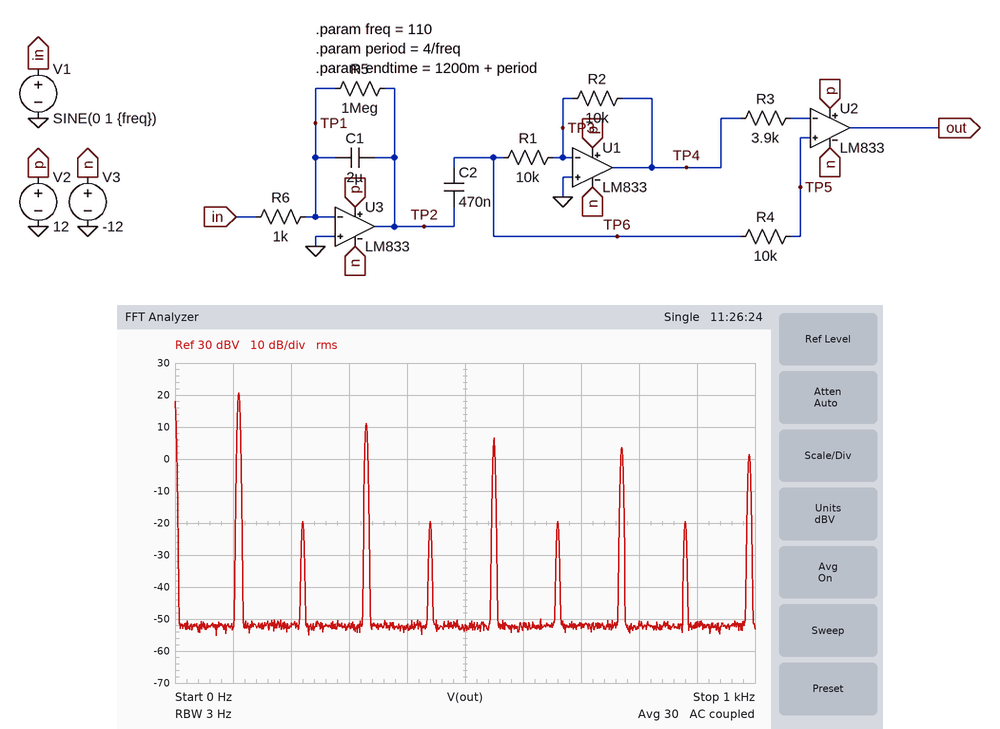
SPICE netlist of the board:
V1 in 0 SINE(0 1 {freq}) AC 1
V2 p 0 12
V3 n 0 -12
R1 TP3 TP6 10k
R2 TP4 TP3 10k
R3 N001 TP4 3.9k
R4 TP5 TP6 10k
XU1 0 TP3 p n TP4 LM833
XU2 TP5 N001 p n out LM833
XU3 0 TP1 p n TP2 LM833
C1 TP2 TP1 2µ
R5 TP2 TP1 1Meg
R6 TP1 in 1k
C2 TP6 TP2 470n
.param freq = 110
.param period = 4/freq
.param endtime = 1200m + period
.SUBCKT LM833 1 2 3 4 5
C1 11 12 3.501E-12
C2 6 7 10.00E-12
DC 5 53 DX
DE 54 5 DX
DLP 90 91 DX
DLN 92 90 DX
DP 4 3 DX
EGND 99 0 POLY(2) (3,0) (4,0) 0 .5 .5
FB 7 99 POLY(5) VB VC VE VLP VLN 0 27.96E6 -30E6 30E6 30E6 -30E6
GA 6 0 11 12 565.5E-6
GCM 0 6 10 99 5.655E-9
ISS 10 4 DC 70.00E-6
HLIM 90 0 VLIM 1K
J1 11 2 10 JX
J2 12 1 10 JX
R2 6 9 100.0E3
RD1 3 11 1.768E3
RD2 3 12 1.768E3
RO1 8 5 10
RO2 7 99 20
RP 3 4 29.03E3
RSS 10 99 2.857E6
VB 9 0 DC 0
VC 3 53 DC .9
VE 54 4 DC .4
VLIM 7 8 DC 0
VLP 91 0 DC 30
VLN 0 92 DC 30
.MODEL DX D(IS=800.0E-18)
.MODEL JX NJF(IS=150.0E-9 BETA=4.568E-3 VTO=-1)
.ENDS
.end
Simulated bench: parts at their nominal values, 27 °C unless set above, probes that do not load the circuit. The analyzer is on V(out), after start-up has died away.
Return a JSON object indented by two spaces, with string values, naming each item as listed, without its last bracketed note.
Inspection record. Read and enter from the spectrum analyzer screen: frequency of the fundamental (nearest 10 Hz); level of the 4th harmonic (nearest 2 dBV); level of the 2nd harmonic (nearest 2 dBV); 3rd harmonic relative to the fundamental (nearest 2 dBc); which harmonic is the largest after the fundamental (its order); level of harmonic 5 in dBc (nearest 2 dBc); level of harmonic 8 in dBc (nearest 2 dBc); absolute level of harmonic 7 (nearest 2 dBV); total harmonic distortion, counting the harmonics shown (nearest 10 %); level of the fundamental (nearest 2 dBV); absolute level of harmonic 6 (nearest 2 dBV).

{
  "frequency of the fundamental": "110 Hz",
  "level of the 4th harmonic": "-20 dBV",
  "level of the 2nd harmonic": "-20 dBV",
  "3rd harmonic relative to the fundamental": "-10 dBc",
  "which harmonic is the largest after the fundamental": "3",
  "level of harmonic 5 in dBc": "-14 dBc",
  "level of harmonic 8 in dBc": "-40 dBc",
  "absolute level of harmonic 7": "4 dBV",
  "total harmonic distortion, counting the harmonics shown": "40 %",
  "level of the fundamental": "20 dBV",
  "absolute level of harmonic 6": "-20 dBV"
}
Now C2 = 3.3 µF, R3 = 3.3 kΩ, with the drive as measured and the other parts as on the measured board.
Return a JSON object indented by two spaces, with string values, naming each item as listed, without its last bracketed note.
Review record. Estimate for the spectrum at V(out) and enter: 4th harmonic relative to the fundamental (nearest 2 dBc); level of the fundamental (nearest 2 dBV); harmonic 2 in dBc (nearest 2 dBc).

{
  "4th harmonic relative to the fundamental": "-34 dBc",
  "level of the fundamental": "20 dBV",
  "harmonic 2 in dBc": "-34 dBc"
}
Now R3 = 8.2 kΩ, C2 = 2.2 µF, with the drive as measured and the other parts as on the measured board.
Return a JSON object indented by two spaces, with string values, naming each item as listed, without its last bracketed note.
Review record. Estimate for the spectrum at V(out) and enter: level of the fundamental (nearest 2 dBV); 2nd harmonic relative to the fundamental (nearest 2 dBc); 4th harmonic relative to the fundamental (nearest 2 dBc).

{
  "level of the fundamental": "20 dBV",
  "2nd harmonic relative to the fundamental": "-36 dBc",
  "4th harmonic relative to the fundamental": "-36 dBc"
}
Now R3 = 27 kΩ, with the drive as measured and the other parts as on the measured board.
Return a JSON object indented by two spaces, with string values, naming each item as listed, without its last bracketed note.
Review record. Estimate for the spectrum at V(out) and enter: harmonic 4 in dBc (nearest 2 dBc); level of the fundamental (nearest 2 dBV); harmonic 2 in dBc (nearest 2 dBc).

{
  "harmonic 4 in dBc": "-46 dBc",
  "level of the fundamental": "20 dBV",
  "harmonic 2 in dBc": "-46 dBc"
}
